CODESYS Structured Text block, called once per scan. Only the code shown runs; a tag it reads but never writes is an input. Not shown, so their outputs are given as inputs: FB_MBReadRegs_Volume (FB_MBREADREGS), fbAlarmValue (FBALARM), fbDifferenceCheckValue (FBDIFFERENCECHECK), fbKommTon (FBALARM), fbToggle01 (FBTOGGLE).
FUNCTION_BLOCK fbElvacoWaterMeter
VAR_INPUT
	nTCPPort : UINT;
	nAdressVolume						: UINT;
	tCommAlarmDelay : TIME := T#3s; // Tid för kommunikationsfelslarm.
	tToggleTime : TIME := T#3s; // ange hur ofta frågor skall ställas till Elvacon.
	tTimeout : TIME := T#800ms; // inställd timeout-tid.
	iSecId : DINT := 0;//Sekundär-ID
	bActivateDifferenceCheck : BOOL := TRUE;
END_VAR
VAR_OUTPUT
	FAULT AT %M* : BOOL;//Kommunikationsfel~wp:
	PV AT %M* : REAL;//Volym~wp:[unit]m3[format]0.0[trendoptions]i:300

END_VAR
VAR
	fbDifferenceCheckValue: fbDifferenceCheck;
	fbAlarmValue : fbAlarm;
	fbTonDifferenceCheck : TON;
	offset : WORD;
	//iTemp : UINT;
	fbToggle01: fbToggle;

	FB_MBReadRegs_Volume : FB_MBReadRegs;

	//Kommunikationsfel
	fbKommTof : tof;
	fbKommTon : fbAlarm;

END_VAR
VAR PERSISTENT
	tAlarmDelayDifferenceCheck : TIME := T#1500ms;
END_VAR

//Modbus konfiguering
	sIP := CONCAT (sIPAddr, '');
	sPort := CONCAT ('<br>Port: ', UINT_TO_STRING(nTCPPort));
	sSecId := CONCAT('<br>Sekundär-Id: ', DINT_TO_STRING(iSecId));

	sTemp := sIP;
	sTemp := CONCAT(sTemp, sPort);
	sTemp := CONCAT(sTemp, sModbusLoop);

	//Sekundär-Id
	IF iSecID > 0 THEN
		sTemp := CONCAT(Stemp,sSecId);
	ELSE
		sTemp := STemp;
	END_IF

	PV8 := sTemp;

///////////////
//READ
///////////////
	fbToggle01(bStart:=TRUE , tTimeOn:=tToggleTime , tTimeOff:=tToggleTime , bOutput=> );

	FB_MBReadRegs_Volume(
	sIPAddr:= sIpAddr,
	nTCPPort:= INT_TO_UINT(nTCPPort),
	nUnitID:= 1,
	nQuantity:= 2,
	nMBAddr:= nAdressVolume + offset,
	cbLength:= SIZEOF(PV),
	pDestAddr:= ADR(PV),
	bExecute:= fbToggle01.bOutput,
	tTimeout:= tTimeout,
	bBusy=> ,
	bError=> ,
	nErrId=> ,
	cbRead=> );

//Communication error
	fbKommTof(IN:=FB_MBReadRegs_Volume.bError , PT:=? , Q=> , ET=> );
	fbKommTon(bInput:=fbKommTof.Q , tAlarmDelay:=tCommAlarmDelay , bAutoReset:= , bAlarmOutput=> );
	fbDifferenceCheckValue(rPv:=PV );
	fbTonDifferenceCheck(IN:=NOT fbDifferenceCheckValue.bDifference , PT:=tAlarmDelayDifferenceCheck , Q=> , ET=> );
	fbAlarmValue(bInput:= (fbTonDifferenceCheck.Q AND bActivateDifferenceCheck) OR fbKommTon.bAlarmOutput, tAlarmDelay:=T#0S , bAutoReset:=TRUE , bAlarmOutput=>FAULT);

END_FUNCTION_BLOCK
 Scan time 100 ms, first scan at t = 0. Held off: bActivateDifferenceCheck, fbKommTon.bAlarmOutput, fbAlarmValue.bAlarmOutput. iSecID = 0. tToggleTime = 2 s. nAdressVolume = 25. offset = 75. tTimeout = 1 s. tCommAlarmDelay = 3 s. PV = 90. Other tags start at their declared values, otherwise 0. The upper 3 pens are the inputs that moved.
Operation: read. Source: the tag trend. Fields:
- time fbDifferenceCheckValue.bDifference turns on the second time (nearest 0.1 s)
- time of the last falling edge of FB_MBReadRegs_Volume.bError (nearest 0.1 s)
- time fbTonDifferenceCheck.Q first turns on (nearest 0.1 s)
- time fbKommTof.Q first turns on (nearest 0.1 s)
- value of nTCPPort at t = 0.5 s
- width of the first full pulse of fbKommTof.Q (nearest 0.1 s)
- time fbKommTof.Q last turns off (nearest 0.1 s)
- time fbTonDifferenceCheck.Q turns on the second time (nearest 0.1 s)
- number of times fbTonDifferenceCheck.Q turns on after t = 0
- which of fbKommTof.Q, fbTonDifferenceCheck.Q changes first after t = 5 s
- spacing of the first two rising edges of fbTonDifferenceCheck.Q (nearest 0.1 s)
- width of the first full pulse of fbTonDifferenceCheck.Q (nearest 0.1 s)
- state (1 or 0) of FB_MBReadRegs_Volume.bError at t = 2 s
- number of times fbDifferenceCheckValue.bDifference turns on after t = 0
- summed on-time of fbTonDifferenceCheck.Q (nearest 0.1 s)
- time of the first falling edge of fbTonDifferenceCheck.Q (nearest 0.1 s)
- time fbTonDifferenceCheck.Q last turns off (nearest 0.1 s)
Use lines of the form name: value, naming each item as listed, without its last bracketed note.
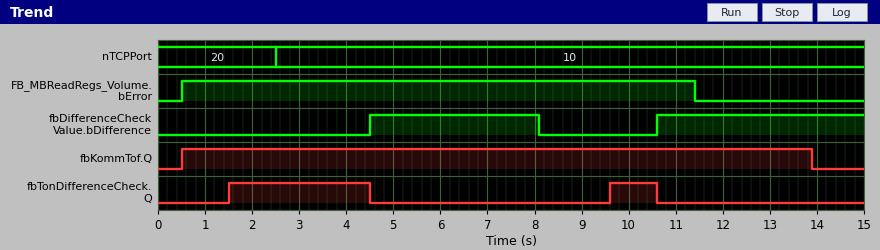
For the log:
time fbDifferenceCheckValue.bDifference turns on the second time: 10.6 s
time of the last falling edge of FB_MBReadRegs_Volume.bError: 11.4 s
time fbTonDifferenceCheck.Q first turns on: 1.5 s
time fbKommTof.Q first turns on: 0.5 s
value of nTCPPort at t = 0.5 s: 20
width of the first full pulse of fbKommTof.Q: 13.4 s
time fbKommTof.Q last turns off: 13.9 s
time fbTonDifferenceCheck.Q turns on the second time: 9.6 s
number of times fbTonDifferenceCheck.Q turns on after t = 0: 2
which of fbKommTof.Q, fbTonDifferenceCheck.Q changes first after t = 5 s: fbTonDifferenceCheck.Q
spacing of the first two rising edges of fbTonDifferenceCheck.Q: 8.1 s
width of the first full pulse of fbTonDifferenceCheck.Q: 3.0 s
state (1 or 0) of FB_MBReadRegs_Volume.bError at t = 2 s: 1
number of times fbDifferenceCheckValue.bDifference turns on after t = 0: 2
summed on-time of fbTonDifferenceCheck.Q: 4.0 s
time of the first falling edge of fbTonDifferenceCheck.Q: 4.5 s
time fbTonDifferenceCheck.Q last turns off: 10.6 s
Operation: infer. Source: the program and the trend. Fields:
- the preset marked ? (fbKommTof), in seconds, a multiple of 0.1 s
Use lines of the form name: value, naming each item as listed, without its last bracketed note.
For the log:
the preset marked ? (fbKommTof), in seconds, a multiple of 0.1 s: 2.5 s
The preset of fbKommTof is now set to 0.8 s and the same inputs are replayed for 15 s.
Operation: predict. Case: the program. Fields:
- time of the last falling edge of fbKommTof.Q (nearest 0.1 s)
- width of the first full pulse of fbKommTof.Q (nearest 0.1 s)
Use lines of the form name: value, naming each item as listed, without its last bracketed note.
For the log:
time of the last falling edge of fbKommTof.Q: 12.2 s
width of the first full pulse of fbKommTof.Q: 11.7 s
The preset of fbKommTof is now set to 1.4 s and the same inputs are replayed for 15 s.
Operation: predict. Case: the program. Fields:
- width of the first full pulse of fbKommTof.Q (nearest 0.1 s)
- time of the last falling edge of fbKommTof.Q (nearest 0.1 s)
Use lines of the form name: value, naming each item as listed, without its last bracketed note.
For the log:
width of the first full pulse of fbKommTof.Q: 12.3 s
time of the last falling edge of fbKommTof.Q: 12.8 s
